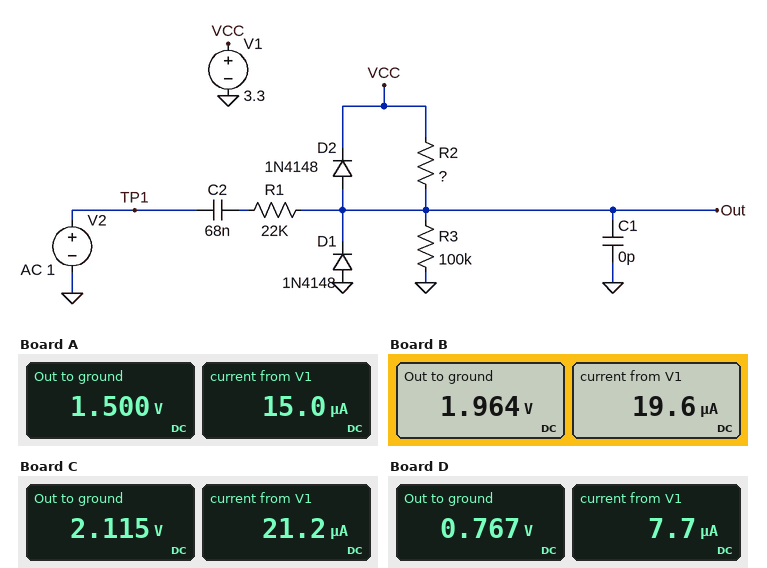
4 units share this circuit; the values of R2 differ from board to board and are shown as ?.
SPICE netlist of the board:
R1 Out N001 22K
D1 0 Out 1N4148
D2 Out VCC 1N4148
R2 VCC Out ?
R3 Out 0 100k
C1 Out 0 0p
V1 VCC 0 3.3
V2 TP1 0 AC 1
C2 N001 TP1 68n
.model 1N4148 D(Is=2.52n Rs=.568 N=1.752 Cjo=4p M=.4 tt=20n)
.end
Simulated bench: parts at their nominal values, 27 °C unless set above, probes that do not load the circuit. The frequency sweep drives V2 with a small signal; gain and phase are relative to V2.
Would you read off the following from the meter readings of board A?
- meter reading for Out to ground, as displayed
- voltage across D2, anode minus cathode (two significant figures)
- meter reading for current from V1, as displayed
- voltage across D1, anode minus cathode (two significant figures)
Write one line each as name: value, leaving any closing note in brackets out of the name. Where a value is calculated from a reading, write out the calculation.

meter reading for Out to ground, as displayed: 1.500 V
voltage across D2, anode minus cathode: 1.5 V - 3.3 V = -1.8 V
meter reading for current from V1, as displayed: 15.0 µA
voltage across D1, anode minus cathode: 0 V - 1.5 V = -1.5 V
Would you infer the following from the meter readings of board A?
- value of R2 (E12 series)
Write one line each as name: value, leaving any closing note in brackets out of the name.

value of R2: 120 kΩ
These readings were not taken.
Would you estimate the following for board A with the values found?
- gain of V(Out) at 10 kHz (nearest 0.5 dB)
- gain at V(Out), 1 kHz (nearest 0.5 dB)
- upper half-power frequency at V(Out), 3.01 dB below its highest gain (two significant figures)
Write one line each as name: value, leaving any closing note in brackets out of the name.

gain of V(Out) at 10 kHz: -3.0 dB
gain at V(Out), 1 kHz: -3.0 dB
upper half-power frequency at V(Out), 3.01 dB below its highest gain: 1.9 MHz
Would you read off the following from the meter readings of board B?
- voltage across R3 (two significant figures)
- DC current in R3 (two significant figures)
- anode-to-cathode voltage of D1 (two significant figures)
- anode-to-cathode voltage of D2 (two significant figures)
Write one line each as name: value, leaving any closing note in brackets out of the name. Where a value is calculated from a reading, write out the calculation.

voltage across R3: 1.964 V = 2.0 V
DC current in R3: (1.964 V) / 100 kΩ = 20 µA
anode-to-cathode voltage of D1: 0 V - 1.964 V = -2.0 V
anode-to-cathode voltage of D2: 1.964 V - 3.3 V = -1.3 V
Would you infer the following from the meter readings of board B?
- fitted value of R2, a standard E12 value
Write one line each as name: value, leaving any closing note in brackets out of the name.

fitted value of R2, a standard E12 value: 68 kΩ
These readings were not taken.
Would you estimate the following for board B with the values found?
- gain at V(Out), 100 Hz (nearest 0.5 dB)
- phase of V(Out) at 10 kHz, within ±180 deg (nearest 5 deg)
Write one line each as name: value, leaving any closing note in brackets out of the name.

gain at V(Out), 100 Hz: -4.5 dB
phase of V(Out) at 10 kHz, within ±180 deg: 0 deg
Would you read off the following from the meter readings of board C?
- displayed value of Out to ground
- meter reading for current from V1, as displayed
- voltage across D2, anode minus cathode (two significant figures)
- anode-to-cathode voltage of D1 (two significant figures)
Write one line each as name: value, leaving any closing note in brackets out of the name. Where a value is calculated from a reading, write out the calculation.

displayed value of Out to ground: 2.115 V
meter reading for current from V1, as displayed: 21.2 µA
voltage across D2, anode minus cathode: 2.115 V - 3.3 V = -1.2 V
anode-to-cathode voltage of D1: 0 V - 2.115 V = -2.1 V
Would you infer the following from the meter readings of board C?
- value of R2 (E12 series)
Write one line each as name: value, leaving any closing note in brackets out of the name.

value of R2: 56 kΩ
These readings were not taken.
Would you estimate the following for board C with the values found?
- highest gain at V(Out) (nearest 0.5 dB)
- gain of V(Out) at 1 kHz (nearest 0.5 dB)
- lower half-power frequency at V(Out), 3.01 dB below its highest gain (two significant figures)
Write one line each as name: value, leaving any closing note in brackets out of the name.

highest gain at V(Out): -4.0 dB
gain of V(Out) at 1 kHz: -4.0 dB
lower half-power frequency at V(Out), 3.01 dB below its highest gain: 40 Hz
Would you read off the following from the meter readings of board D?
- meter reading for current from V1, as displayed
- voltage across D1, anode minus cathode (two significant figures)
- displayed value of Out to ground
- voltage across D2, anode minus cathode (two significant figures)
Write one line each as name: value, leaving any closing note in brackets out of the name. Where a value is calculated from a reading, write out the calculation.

meter reading for current from V1, as displayed: 7.7 µA
voltage across D1, anode minus cathode: 0 V - 767 mV = -770 mV
displayed value of Out to ground: 0.767 V
voltage across D2, anode minus cathode: 767 mV - 3.3 V = -2.5 V
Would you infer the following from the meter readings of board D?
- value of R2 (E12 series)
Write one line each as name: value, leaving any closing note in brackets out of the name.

value of R2: 330 kΩ
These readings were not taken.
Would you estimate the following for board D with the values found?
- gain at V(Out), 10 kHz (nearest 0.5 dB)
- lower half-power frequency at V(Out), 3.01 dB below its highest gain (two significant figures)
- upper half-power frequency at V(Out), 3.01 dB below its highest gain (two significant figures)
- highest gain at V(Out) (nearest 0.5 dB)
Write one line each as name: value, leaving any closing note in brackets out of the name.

gain at V(Out), 10 kHz: -2.0 dB
lower half-power frequency at V(Out), 3.01 dB below its highest gain: 24 Hz
upper half-power frequency at V(Out), 3.01 dB below its highest gain: 1.7 MHz
highest gain at V(Out): -2.0 dB
